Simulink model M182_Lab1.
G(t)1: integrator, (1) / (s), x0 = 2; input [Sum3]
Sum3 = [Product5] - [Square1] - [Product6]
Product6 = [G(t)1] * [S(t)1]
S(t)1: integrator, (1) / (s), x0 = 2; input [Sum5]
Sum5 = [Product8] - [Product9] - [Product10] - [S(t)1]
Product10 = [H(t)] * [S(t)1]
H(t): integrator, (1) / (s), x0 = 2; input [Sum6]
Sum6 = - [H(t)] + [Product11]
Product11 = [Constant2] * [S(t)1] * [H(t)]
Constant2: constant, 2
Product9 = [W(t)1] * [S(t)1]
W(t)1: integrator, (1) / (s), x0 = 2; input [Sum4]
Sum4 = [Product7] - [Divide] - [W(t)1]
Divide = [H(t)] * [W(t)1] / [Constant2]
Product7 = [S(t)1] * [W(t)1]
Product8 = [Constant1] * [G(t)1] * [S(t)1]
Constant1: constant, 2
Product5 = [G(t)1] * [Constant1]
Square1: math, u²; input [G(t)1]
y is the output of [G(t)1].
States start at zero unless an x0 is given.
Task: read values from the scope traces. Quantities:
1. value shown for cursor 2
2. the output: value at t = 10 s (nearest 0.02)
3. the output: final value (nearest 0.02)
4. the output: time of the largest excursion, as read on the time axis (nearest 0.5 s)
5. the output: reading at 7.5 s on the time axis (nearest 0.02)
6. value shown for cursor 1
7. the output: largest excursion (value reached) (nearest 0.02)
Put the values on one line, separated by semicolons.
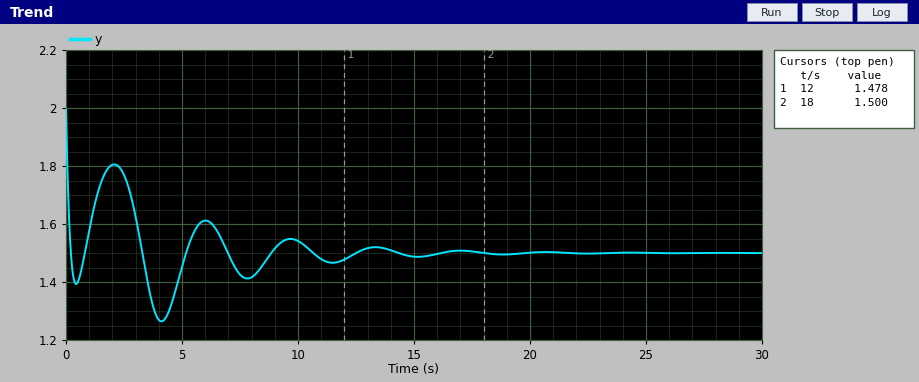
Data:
1.500; 1.54; 1.50; 4.0 s; 1.42; 1.478; 1.26
